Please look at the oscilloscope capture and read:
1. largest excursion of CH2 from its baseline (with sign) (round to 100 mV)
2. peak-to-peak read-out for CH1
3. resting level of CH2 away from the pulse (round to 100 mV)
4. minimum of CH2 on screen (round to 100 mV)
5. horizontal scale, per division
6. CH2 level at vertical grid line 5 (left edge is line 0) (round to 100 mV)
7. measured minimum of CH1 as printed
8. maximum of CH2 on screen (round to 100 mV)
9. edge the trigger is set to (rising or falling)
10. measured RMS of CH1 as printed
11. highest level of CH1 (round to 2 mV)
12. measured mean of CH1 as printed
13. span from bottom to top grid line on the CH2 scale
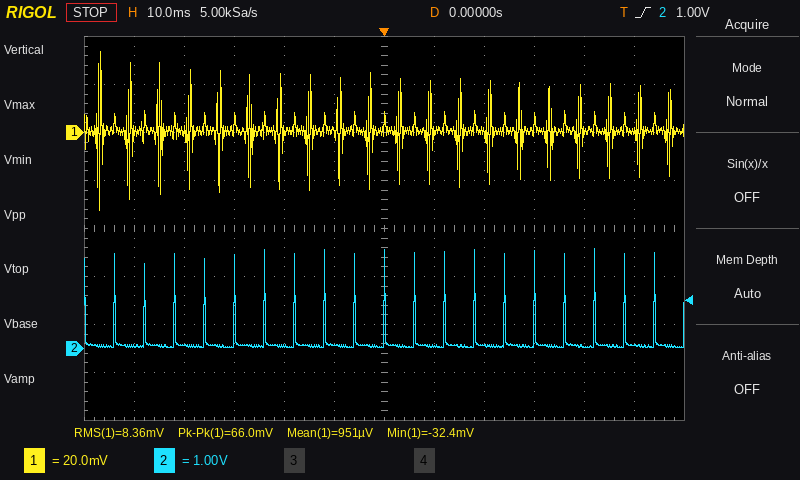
+2.0 V
66.0 mV
100 mV
0.0 V
10 ms
100 mV
-32.4 mV
2.1 V
rising
8.36 mV
34 mV
951 µV
8 V
